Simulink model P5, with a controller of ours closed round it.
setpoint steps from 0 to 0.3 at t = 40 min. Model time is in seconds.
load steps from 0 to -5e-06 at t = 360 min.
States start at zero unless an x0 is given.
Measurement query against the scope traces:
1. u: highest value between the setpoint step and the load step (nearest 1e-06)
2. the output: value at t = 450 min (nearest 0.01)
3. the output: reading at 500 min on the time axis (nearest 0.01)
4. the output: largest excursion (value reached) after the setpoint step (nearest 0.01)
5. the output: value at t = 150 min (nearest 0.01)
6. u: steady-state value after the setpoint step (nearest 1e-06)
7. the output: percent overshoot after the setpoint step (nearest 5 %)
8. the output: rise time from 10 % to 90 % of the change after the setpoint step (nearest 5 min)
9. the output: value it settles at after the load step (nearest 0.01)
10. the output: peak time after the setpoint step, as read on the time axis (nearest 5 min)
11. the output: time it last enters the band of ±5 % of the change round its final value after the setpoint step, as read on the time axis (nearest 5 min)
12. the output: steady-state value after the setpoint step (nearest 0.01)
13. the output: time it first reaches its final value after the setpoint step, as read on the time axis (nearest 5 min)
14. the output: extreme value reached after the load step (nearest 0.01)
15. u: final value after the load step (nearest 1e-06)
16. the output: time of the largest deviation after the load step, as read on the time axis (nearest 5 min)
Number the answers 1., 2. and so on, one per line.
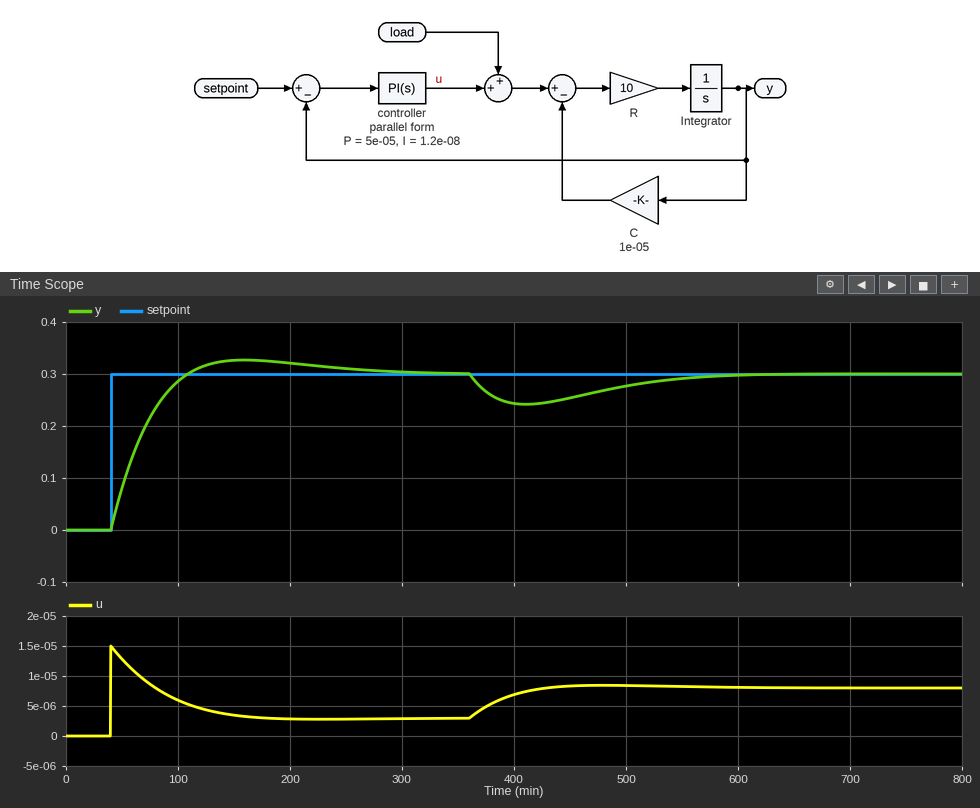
1. 0.000015
2. 0.25
3. 0.28
4. 0.33
5. 0.33
6. 0.000003
7. 10 %
8. 50 min
9. 0.30
10. 160 min
11. 225 min
12. 0.30
13. 110 min
14. 0.24
15. 0.000008
16. 410 min
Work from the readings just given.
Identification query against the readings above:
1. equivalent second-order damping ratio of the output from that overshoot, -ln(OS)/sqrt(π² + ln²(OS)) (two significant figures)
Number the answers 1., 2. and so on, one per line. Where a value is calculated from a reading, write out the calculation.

1. ln(0.1) = -2.303; 2.303 / sqrt(9.870 + 5.302) = 0.59
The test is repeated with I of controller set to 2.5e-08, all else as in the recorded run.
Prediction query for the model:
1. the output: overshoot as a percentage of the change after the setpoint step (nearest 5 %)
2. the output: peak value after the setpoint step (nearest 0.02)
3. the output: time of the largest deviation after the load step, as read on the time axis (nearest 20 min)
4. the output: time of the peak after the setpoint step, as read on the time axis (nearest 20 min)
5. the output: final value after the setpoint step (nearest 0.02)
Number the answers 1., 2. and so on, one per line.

1. 20 %
2. 0.36
3. 400 min
4. 120 min
5. 0.30
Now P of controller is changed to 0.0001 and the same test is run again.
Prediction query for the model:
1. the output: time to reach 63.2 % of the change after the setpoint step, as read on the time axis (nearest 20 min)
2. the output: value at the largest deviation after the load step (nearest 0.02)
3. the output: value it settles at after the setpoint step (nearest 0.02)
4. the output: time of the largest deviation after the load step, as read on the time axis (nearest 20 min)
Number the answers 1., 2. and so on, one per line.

1. 60 min
2. 0.26
3. 0.30
4. 400 min
